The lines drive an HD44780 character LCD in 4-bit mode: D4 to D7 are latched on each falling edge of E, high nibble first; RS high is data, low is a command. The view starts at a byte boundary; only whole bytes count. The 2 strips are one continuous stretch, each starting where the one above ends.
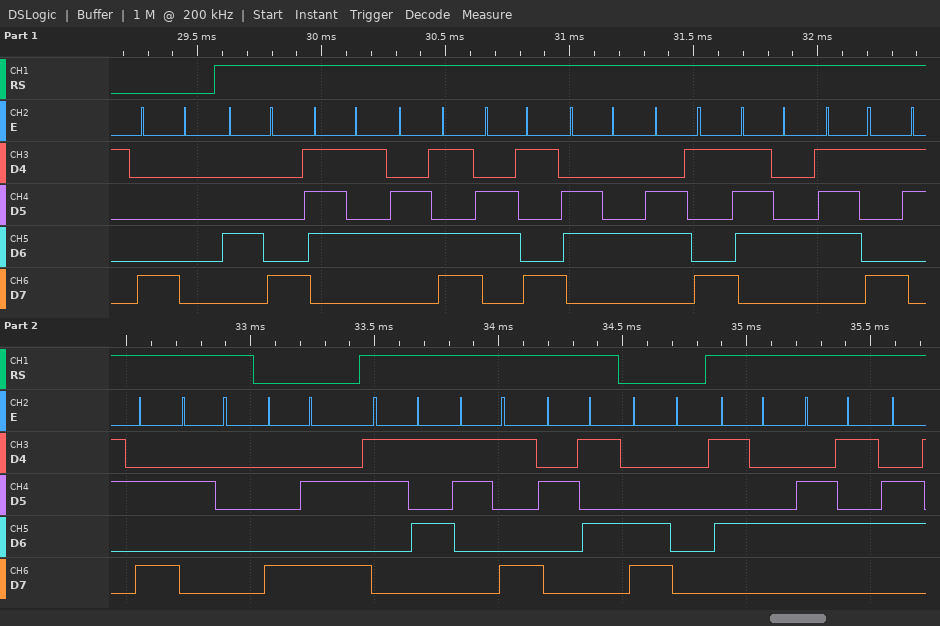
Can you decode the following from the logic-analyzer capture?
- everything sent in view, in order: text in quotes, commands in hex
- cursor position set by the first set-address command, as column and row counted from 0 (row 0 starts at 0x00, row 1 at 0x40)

0x80 "Humidity: " 0x8A "59%" 0xC0 "Te"
column 0, row 0
